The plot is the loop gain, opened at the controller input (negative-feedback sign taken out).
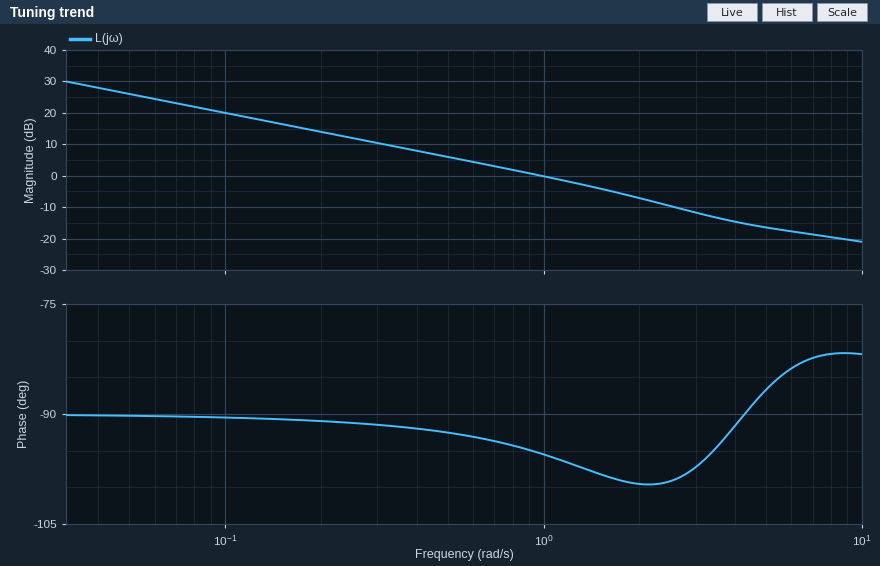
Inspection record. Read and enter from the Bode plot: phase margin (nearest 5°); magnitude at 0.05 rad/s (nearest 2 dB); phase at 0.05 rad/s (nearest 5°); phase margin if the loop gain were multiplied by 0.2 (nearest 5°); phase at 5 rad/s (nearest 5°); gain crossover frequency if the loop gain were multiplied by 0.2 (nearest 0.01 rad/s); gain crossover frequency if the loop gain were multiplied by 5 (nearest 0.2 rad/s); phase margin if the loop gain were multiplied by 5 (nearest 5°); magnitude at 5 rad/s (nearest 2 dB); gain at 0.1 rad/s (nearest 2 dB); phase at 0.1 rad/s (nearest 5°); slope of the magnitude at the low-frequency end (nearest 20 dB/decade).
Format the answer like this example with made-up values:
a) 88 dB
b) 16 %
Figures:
a) 85°
b) 26 dB
c) -90°
d) 90°
e) -85°
f) 0.20 rad/s
g) 3.8 rad/s
h) 85°
i) -16 dB
j) 20 dB
k) -90°
l) -20 dB/decade
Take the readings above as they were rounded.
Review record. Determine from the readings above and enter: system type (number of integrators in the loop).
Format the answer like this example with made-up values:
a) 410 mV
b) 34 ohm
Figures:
a) 1
